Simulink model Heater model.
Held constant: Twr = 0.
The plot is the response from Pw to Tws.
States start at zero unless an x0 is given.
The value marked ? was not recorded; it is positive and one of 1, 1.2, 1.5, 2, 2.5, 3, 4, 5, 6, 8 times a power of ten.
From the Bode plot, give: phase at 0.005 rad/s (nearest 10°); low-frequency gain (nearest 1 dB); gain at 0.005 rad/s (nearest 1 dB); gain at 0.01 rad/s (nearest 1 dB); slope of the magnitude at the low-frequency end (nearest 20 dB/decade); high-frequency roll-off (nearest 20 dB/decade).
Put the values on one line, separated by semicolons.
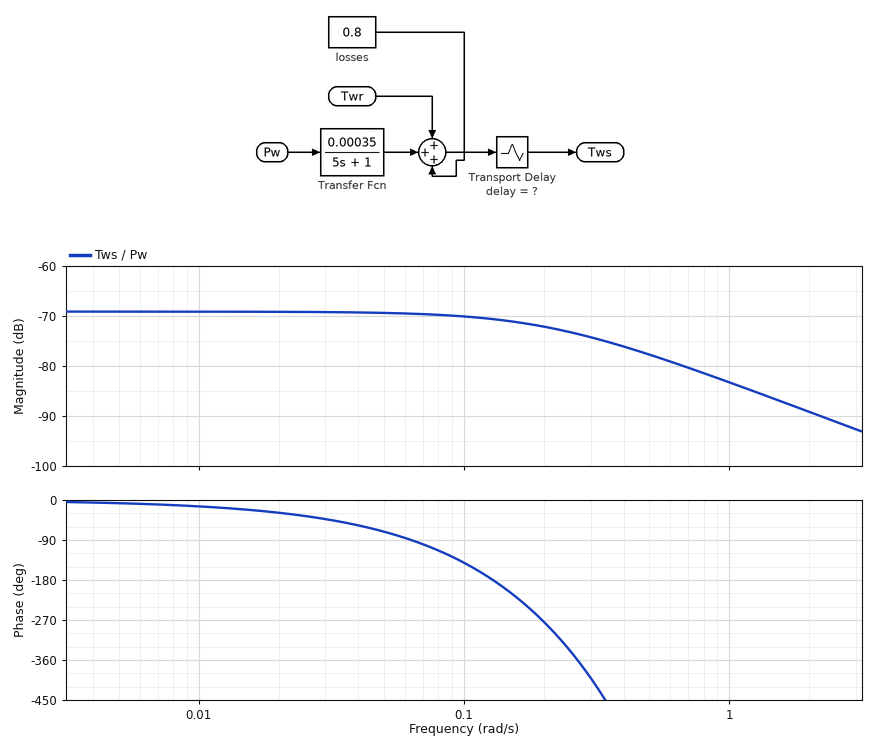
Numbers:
-10°; -69 dB; -69 dB; -69 dB; 0 dB/decade; -20 dB/decade
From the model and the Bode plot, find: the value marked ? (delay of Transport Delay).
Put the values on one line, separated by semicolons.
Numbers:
20
